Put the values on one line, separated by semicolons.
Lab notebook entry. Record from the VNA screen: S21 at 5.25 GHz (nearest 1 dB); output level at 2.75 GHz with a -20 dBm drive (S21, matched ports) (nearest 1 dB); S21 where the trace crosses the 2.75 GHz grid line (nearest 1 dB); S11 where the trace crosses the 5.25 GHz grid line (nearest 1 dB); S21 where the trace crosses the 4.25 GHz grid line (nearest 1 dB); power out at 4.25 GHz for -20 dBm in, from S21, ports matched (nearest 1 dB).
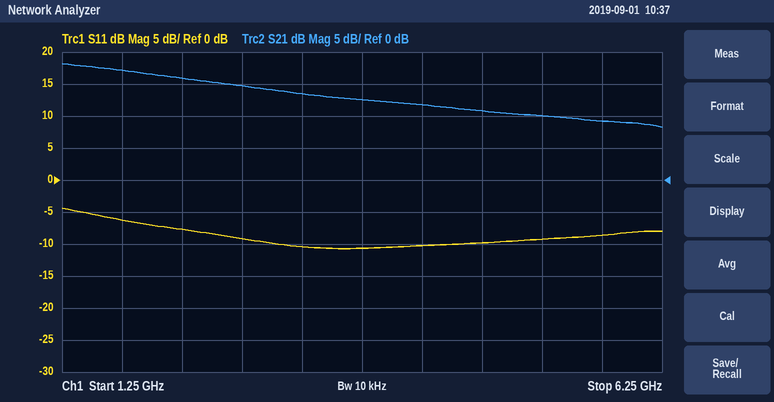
10 dB; -5 dBm; 15 dB; -9 dB; 12 dB; -8 dBm
